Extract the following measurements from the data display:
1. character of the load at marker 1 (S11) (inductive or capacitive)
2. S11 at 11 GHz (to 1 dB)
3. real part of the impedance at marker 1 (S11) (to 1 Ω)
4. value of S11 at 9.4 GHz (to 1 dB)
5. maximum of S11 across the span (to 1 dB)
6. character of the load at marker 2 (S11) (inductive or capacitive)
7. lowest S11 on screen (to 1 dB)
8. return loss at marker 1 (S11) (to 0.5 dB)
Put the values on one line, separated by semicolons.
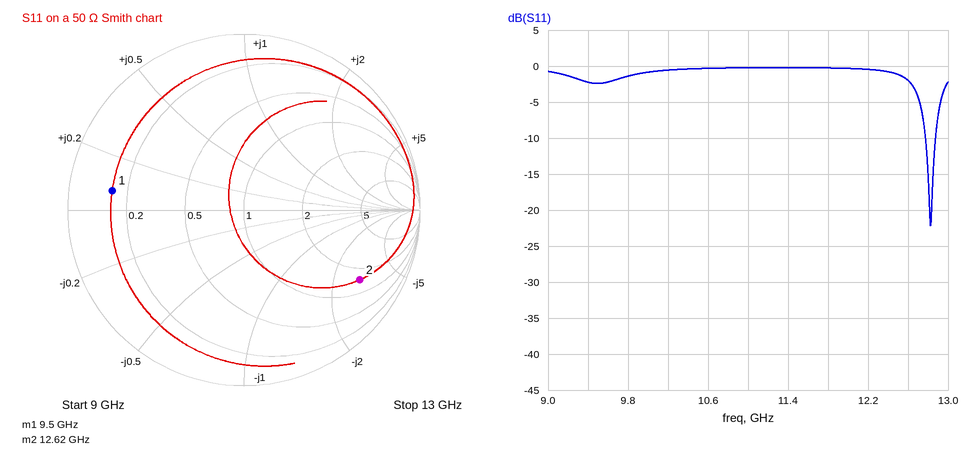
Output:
inductive; 0 dB; 7 Ω; -2 dB; 0 dB; capacitive; -22 dB; 2.5 dB
